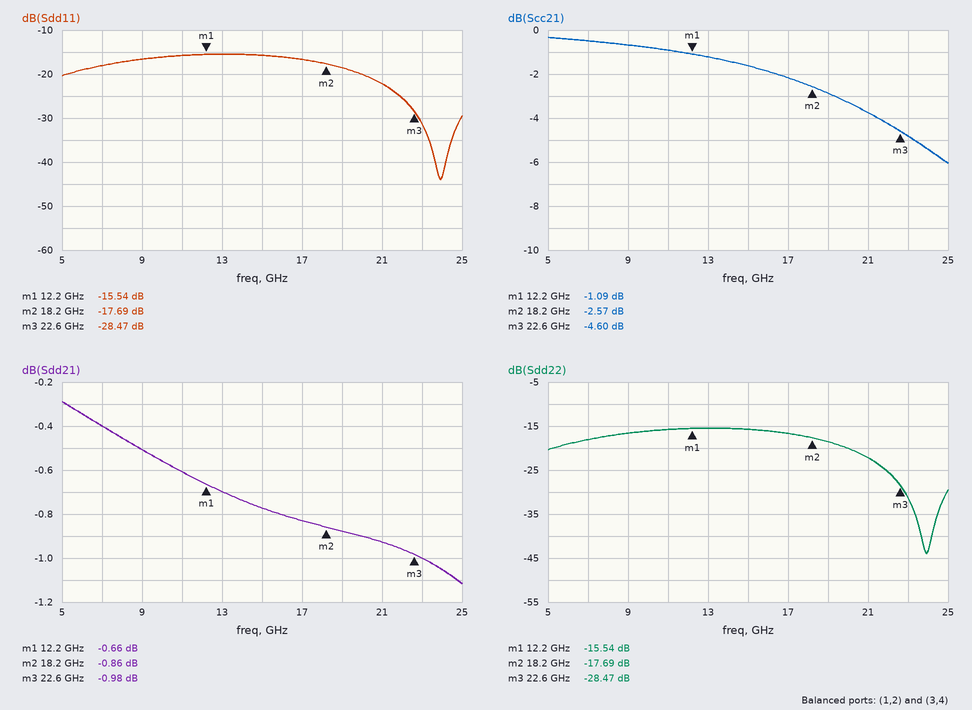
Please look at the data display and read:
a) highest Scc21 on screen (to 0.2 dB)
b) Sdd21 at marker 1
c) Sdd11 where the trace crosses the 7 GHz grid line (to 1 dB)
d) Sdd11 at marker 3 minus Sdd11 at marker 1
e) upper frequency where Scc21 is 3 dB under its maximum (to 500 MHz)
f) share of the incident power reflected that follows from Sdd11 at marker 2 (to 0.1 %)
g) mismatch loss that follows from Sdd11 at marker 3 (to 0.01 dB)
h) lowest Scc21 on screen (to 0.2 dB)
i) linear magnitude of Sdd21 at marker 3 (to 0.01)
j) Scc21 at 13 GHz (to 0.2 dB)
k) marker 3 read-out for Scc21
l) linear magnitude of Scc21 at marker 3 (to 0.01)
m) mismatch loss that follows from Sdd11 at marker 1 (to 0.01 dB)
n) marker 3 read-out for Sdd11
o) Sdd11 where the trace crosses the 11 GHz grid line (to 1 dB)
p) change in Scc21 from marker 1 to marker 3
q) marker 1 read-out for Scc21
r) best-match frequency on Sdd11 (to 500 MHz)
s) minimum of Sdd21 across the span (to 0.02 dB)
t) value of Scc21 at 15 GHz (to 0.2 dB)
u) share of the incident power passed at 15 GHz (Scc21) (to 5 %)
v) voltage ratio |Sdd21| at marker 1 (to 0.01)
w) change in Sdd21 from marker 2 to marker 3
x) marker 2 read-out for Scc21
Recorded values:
-0.4 dB
-0.66 dB
-18 dB
-12.93 dB
20.0 GHz
1.7 %
0.01 dB
-6.0 dB
0.89
-1.2 dB
-4.60 dB
0.59
0.12 dB
-28.47 dB
-16 dB
-3.51 dB
-1.09 dB
24.0 GHz
-1.12 dB
-1.6 dB
70 %
0.93
-0.12 dB
-2.57 dB
